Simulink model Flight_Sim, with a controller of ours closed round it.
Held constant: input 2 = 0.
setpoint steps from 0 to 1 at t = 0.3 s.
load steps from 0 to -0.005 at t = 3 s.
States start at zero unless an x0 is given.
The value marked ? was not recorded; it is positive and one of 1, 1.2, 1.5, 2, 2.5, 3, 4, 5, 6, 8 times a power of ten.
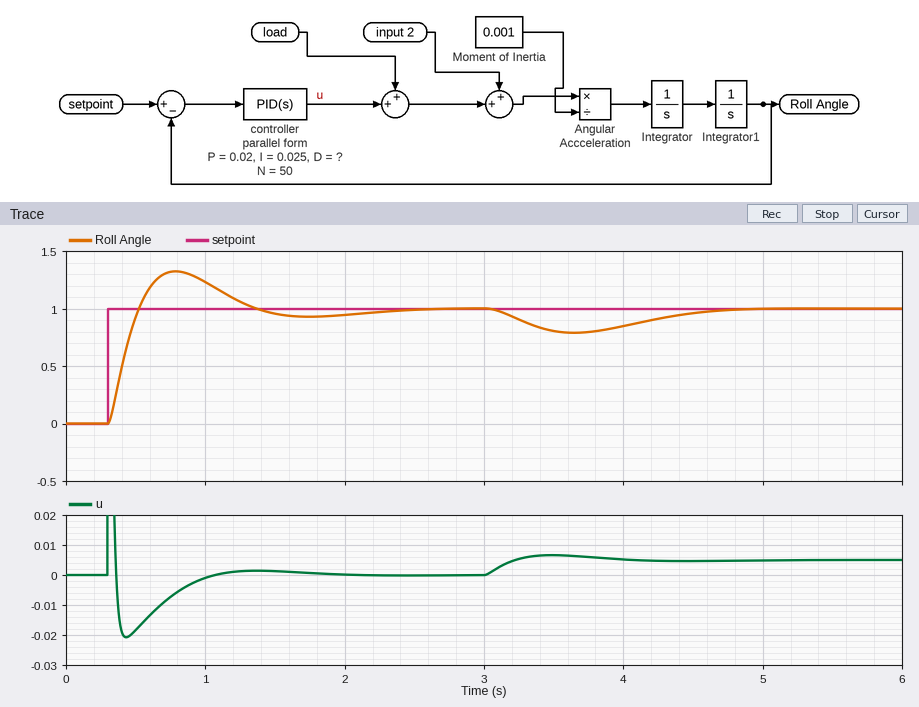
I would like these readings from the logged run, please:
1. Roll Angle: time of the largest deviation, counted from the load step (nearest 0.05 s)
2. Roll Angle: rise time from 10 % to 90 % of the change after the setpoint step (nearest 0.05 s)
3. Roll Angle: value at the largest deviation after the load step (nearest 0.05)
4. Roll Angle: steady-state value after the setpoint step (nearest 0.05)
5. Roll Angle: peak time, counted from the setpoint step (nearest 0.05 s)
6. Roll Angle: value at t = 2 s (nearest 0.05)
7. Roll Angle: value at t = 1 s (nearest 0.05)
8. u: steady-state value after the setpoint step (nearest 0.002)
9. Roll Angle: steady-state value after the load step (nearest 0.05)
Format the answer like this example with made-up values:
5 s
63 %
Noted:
0.65 s
0.15 s
0.80
1.00
0.50 s
0.95
1.25
0.000
1.00
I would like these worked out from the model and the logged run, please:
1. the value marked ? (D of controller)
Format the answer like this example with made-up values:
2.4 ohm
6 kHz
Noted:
0.006
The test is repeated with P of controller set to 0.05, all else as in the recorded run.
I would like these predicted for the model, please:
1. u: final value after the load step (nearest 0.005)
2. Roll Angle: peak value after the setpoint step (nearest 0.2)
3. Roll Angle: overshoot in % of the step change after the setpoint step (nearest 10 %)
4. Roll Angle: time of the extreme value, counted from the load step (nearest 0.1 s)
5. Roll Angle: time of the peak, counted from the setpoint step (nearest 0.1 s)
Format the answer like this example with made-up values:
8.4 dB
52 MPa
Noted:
0.005
1.4
40 %
0.4 s
0.3 s
